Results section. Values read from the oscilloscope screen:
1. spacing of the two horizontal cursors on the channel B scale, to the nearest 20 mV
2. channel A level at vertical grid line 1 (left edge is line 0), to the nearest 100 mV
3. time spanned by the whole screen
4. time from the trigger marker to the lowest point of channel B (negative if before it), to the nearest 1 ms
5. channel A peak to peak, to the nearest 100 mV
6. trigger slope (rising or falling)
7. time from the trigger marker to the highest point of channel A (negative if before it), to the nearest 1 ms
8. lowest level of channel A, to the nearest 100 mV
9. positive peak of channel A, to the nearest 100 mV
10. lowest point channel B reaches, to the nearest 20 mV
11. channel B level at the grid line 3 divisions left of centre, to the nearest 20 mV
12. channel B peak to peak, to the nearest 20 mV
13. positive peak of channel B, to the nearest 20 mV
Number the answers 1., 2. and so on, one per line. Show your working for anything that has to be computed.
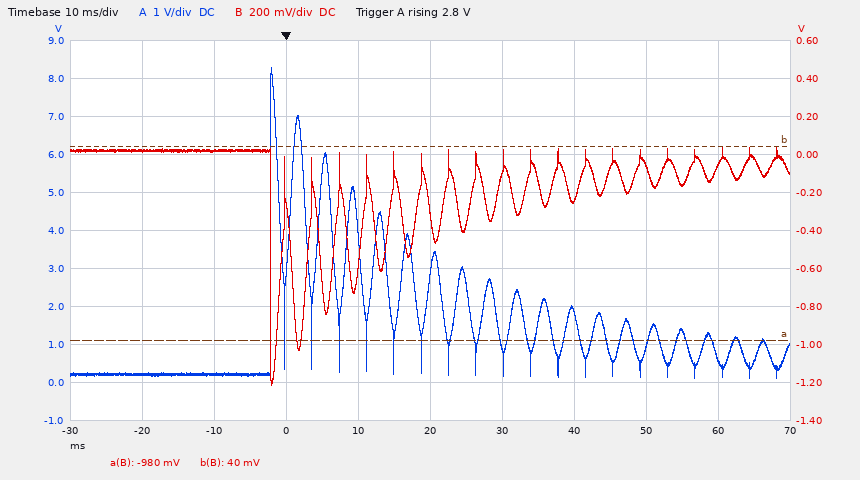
1. 1.02 V
2. 200 mV
3. 100 ms
4. -2 ms
5. 8.3 V − (100 mV) = 8.2 V
6. rising
7. -2 ms
8. 100 mV
9. 8.3 V
10. -1.22 V
11. 20 mV
12. 40 mV − (-1.22 V) = 1.26 V
13. 40 mV
